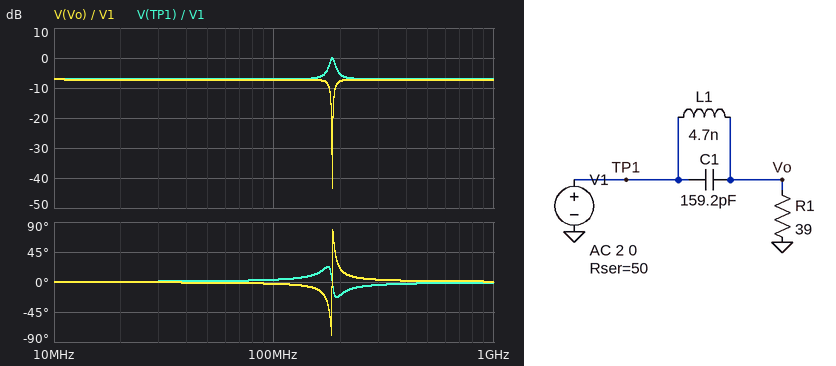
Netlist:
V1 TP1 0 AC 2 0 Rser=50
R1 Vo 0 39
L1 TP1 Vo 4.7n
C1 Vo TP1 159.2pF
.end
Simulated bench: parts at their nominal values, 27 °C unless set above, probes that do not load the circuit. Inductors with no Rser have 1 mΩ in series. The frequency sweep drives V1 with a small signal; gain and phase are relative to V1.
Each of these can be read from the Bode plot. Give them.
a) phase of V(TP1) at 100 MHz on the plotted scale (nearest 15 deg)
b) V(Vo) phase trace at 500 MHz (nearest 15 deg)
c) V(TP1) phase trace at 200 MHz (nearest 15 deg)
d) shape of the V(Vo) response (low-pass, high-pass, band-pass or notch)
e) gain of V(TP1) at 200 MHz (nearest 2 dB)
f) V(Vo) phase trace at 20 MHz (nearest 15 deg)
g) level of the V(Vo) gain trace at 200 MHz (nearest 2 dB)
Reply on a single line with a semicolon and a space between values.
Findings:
0 deg; 0 deg; -15 deg; notch; -6 dB; 0 deg; -8 dB
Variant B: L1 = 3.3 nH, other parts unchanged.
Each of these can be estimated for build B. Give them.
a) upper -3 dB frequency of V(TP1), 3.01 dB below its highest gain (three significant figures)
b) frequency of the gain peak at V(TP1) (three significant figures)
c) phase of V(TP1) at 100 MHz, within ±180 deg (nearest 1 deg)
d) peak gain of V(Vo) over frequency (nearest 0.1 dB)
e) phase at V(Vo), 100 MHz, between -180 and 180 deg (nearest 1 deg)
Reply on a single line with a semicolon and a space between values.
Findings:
227 MHz; 220 MHz; 2 deg; -7.2 dB; -2 deg
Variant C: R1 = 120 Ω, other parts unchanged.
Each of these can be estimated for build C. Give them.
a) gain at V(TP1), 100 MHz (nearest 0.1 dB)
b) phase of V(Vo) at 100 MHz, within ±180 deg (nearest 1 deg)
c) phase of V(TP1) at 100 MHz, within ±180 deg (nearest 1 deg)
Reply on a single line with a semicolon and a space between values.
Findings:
-3.0 dB; -1 deg; 1 deg
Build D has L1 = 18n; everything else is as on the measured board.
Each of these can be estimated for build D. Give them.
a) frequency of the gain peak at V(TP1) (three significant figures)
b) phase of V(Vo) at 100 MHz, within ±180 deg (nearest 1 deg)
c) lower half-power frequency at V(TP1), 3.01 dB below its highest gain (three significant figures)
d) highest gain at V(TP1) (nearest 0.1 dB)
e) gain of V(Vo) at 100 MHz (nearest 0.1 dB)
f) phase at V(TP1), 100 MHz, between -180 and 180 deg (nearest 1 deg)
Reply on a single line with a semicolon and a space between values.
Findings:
94.0 MHz; 44 deg; 87.1 MHz; 0 dB; -10.0 dB; -22 deg
